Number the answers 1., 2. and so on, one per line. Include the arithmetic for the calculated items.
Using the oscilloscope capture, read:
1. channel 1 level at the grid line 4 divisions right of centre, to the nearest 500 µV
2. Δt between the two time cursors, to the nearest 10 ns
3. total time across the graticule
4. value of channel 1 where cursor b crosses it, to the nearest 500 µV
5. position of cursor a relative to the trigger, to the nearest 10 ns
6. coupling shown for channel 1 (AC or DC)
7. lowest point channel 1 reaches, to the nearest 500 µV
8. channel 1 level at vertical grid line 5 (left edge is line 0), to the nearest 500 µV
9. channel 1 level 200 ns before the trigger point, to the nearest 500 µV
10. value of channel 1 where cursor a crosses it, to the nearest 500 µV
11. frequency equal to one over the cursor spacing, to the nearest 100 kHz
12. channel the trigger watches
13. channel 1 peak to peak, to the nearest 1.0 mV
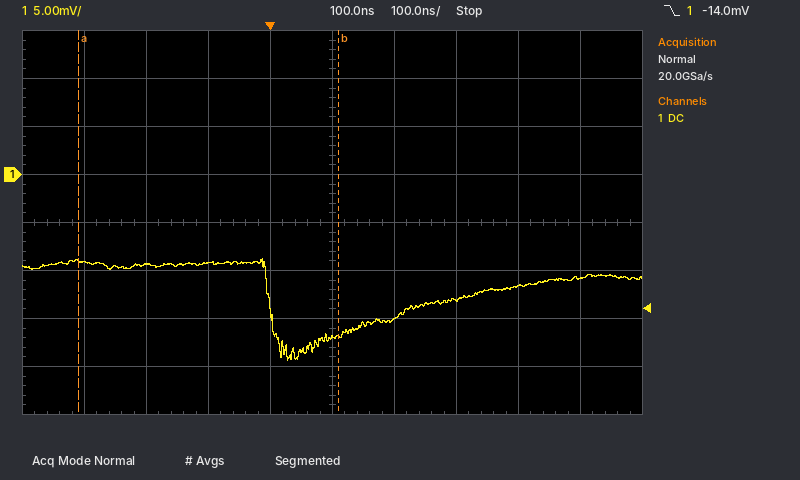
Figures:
1. -11.0 mV
2. 420 ns
3. 1 µs
4. -17.0 mV
5. -310 ns
6. DC
7. -19.5 mV
8. -17.0 mV
9. -9.5 mV
10. -9.0 mV
11. 1 / 420 ns ≈ 2.4 MHz
12. channel 1
13. 11.0 mV
